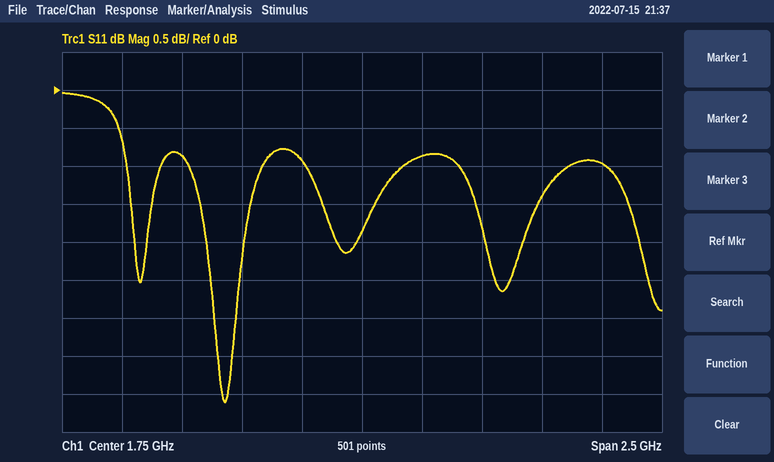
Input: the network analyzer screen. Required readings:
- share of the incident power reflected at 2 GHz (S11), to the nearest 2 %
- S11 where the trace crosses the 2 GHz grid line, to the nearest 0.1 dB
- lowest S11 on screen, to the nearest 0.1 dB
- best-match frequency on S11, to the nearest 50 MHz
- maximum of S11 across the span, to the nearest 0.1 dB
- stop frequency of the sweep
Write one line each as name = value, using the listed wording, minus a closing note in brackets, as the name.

share of the incident power reflected at 2 GHz (S11), to the nearest 2 % = 82 %
S11 where the trace crosses the 2 GHz grid line, to the nearest 0.1 dB = -0.9 dB
lowest S11 on screen, to the nearest 0.1 dB = -4.1 dB
best-match frequency on S11, to the nearest 50 MHz = 1.20 GHz
maximum of S11 across the span, to the nearest 0.1 dB = 0.0 dB
stop frequency of the sweep = 3 GHz
